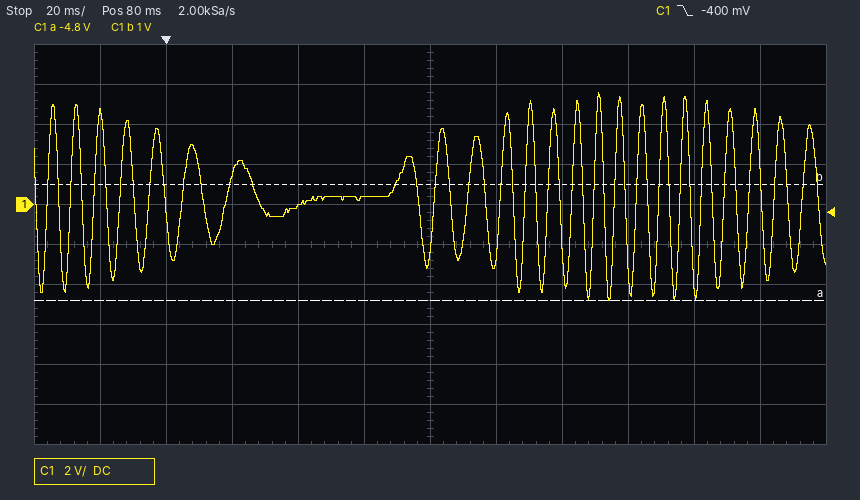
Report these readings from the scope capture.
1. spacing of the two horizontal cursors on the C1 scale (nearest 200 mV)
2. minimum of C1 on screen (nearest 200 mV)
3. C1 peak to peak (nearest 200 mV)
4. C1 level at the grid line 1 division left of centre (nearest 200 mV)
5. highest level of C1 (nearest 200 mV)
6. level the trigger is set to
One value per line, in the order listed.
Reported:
5.8 V
-4.8 V
10.4 V
400 mV
5.6 V
-400 mV
